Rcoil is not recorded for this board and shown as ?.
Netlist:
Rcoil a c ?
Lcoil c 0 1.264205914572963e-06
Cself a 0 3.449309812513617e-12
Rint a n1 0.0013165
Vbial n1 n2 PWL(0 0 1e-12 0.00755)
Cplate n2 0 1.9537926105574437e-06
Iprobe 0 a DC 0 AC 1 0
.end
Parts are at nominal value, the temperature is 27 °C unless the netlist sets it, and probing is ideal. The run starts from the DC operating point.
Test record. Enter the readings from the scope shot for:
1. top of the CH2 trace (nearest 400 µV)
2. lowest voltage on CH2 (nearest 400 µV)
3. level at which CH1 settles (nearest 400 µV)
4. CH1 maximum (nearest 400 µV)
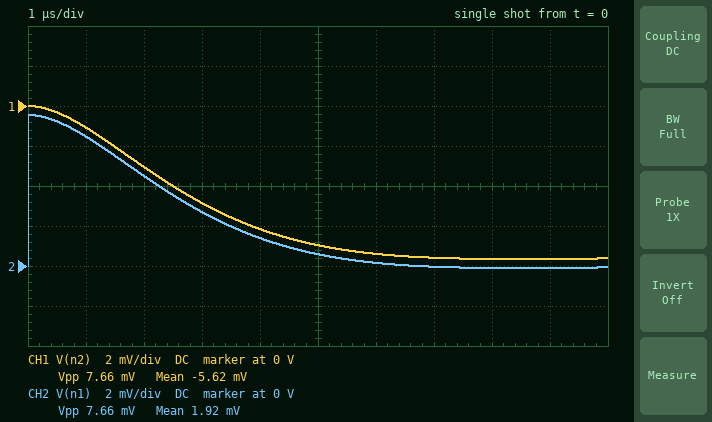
7.6 mV
0 V
-7.6 mV
0 V
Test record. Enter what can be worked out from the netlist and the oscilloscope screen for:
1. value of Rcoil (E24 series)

1.3 Ω
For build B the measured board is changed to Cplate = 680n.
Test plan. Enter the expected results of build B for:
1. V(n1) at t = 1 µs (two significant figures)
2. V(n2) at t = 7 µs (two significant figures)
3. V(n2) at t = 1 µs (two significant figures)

4.6 mV
-7.3 mV
-2.9 mV
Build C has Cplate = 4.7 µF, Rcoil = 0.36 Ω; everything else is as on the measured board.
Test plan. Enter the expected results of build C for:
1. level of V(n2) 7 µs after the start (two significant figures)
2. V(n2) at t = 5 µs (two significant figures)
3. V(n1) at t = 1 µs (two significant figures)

-9.6 mV
-7.5 mV
7.0 mV
